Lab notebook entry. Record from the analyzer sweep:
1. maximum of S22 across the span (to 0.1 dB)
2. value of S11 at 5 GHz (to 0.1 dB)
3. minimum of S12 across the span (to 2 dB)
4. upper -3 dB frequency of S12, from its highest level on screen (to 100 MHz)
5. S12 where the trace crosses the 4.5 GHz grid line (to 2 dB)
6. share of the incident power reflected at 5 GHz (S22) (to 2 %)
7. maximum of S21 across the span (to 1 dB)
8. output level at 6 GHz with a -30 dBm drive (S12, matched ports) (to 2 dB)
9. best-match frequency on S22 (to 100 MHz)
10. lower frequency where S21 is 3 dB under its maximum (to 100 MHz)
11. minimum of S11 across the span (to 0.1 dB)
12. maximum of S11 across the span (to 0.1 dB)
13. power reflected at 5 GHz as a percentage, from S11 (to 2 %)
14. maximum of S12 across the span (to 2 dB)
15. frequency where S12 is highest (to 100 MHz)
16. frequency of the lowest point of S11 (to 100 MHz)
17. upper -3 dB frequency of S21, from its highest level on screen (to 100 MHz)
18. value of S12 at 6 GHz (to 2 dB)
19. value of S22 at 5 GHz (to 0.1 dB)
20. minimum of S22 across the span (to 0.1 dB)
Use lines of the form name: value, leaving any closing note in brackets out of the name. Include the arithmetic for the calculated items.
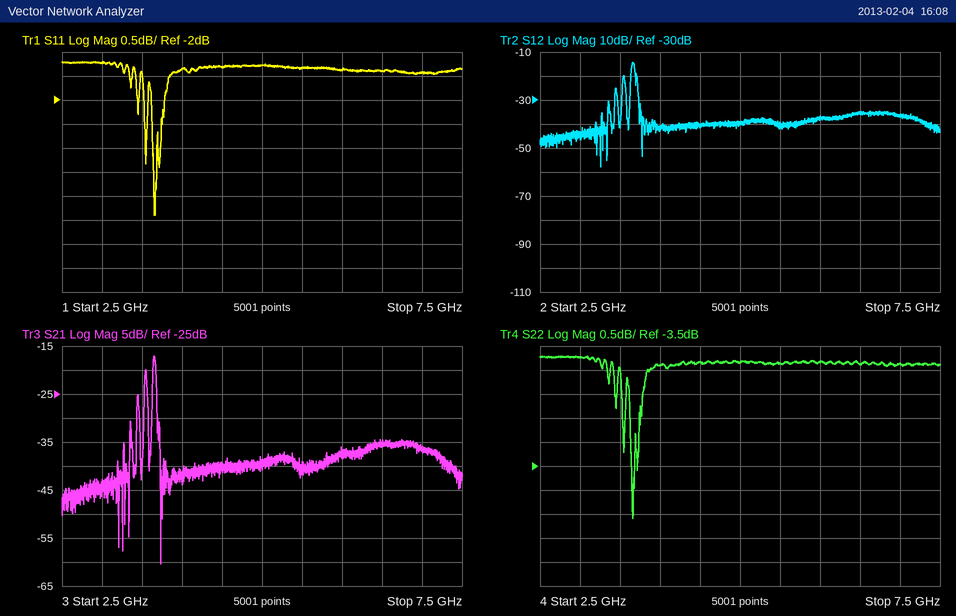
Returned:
maximum of S22 across the span: -1.2 dB
value of S11 at 5 GHz: -1.3 dB
minimum of S12 across the span: -58 dB
upper -3 dB frequency of S12, from its highest level on screen: 3.7 GHz
S12 where the trace crosses the 4.5 GHz grid line: -40 dB
share of the incident power reflected at 5 GHz (S22): 10^(-1.3/10) ≈ 74 %
maximum of S21 across the span: -17 dB
output level at 6 GHz with a -30 dBm drive (S12, matched ports): -30 dBm + (-38 dB) = -68 dBm
best-match frequency on S22: 3.7 GHz
lower frequency where S21 is 3 dB under its maximum: 3.6 GHz
minimum of S11 across the span: -4.4 dB
maximum of S11 across the span: -1.2 dB
power reflected at 5 GHz as a percentage, from S11: 10^(-1.3/10) ≈ 74 %
maximum of S12 across the span: -14 dB
frequency where S12 is highest: 3.7 GHz
frequency of the lowest point of S11: 3.7 GHz
upper -3 dB frequency of S21, from its highest level on screen: 3.7 GHz
value of S12 at 6 GHz: -38 dB
value of S22 at 5 GHz: -1.3 dB
minimum of S22 across the span: -4.6 dB
